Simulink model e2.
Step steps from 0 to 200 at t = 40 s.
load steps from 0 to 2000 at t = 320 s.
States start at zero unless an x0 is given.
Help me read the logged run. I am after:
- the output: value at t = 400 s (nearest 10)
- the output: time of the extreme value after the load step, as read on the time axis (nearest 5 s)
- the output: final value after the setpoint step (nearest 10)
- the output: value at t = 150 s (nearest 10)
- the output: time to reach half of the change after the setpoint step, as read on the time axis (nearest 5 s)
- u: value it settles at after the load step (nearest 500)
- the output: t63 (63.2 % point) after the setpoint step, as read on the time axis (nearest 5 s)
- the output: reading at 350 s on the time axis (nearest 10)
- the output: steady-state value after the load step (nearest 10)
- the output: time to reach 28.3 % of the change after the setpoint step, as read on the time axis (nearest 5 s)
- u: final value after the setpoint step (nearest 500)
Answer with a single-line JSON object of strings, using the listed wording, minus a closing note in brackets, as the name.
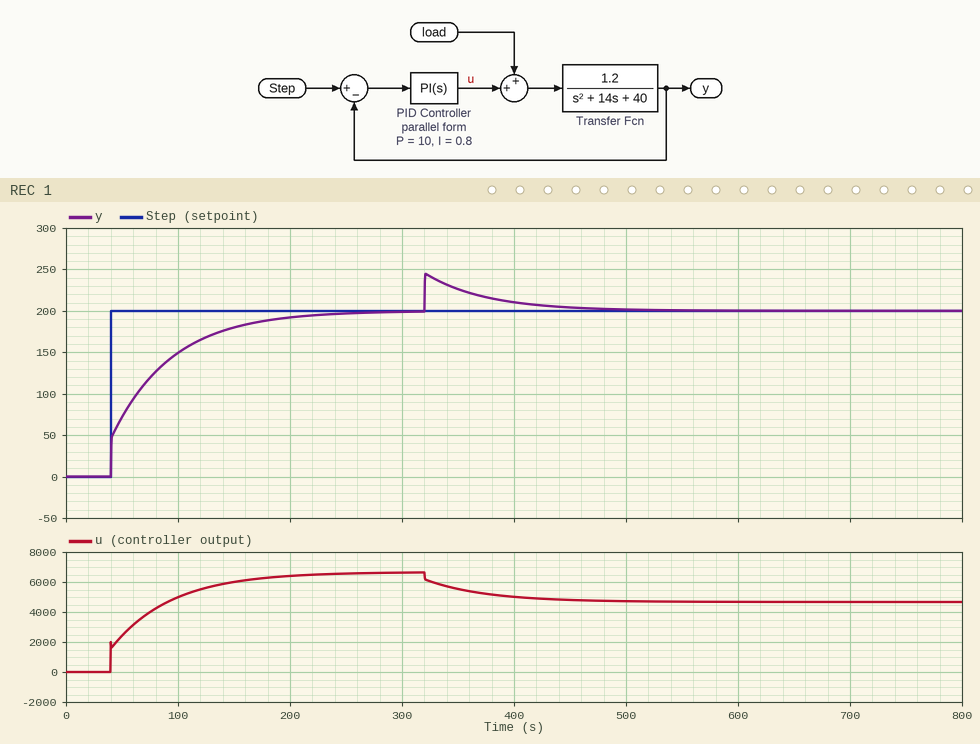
{"the output: value at t = 400 s": "210", "the output: time of the extreme value after the load step, as read on the time axis": "320 s", "the output: final value after the setpoint step": "200", "the output: value at t = 150 s": "180", "the output: time to reach half of the change after the setpoint step, as read on the time axis": "65 s", "u: value it settles at after the load step": "4500", "the output: t63 (63.2 % point) after the setpoint step, as read on the time axis": "80 s", "the output: reading at 350 s on the time axis": "230", "the output: steady-state value after the load step": "200", "the output: time to reach 28.3 % of the change after the setpoint step, as read on the time axis": "45 s", "u: final value after the setpoint step": "6500"}
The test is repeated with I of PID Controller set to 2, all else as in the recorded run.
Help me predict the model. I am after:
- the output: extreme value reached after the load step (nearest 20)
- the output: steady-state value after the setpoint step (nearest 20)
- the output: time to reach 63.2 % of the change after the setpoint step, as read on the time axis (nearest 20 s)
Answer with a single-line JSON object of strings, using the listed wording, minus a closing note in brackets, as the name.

{"the output: extreme value reached after the load step": "240", "the output: steady-state value after the setpoint step": "200", "the output: time to reach 63.2 % of the change after the setpoint step, as read on the time axis": "60 s"}
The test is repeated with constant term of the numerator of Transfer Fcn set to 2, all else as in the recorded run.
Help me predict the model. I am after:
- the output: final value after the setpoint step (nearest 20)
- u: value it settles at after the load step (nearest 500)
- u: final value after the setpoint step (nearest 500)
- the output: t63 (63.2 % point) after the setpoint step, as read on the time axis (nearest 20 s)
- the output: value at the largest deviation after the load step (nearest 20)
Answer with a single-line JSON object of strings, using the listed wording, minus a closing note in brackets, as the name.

{"the output: final value after the setpoint step": "200", "u: value it settles at after the load step": "2000", "u: final value after the setpoint step": "4000", "the output: t63 (63.2 % point) after the setpoint step, as read on the time axis": "60 s", "the output: value at the largest deviation after the load step": "260"}
